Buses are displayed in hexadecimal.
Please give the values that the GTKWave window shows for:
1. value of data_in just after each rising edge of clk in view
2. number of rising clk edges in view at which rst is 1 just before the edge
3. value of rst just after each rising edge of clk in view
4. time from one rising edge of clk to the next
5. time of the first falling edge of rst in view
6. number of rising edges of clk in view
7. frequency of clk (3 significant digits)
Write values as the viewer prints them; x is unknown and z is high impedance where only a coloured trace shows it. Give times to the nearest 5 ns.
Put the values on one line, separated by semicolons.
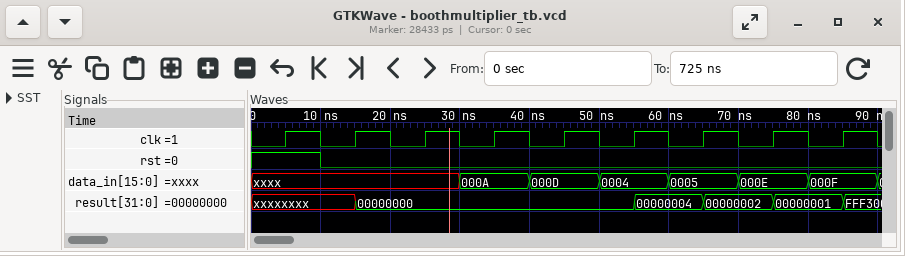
xxxx, xxxx, xxxx, 000A, 000D, 0004, 0005, 000E, 000F; 1; 1 0 0 0 0 0 0 0 0; 10 ns; 10 ns; 9; 100 MHz
